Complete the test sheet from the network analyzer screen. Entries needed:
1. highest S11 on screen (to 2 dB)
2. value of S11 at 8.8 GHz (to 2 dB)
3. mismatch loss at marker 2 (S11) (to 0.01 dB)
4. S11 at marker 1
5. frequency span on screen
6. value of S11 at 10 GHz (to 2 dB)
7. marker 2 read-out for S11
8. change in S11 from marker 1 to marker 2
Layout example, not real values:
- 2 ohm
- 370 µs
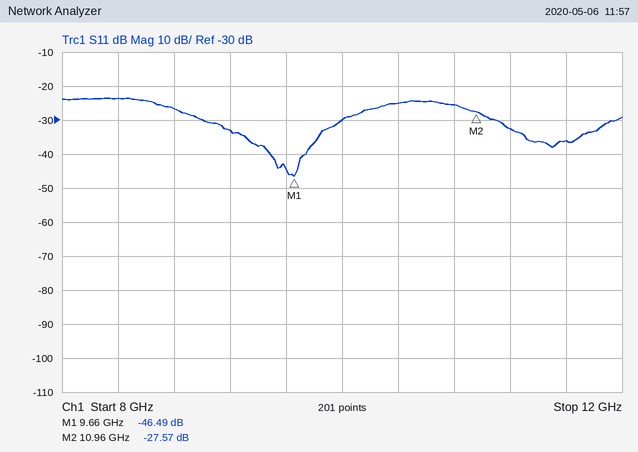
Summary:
- -24 dB
- -26 dB
- 0.01 dB
- -46.49 dB
- 4 GHz
- -30 dB
- -27.57 dB
- 18.92 dB
